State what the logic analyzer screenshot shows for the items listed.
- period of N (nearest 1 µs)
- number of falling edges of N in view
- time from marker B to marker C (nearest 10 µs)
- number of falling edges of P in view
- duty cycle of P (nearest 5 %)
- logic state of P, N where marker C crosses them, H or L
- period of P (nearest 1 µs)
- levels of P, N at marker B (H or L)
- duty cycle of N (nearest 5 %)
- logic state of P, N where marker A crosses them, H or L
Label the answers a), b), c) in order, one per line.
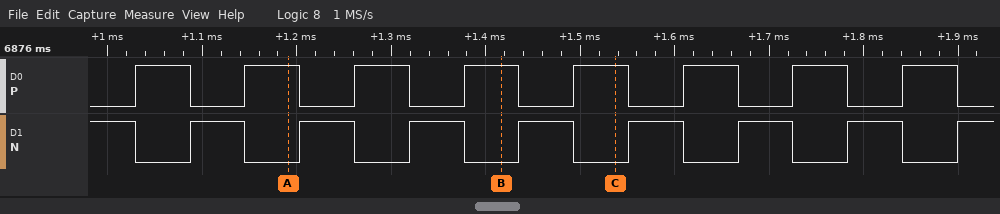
a) 116 µs
b) 8
c) 120 µs
d) 8
e) 50 %
f) P=H, N=L
g) 116 µs
h) P=H, N=L
i) 50 %
j) P=H, N=L
